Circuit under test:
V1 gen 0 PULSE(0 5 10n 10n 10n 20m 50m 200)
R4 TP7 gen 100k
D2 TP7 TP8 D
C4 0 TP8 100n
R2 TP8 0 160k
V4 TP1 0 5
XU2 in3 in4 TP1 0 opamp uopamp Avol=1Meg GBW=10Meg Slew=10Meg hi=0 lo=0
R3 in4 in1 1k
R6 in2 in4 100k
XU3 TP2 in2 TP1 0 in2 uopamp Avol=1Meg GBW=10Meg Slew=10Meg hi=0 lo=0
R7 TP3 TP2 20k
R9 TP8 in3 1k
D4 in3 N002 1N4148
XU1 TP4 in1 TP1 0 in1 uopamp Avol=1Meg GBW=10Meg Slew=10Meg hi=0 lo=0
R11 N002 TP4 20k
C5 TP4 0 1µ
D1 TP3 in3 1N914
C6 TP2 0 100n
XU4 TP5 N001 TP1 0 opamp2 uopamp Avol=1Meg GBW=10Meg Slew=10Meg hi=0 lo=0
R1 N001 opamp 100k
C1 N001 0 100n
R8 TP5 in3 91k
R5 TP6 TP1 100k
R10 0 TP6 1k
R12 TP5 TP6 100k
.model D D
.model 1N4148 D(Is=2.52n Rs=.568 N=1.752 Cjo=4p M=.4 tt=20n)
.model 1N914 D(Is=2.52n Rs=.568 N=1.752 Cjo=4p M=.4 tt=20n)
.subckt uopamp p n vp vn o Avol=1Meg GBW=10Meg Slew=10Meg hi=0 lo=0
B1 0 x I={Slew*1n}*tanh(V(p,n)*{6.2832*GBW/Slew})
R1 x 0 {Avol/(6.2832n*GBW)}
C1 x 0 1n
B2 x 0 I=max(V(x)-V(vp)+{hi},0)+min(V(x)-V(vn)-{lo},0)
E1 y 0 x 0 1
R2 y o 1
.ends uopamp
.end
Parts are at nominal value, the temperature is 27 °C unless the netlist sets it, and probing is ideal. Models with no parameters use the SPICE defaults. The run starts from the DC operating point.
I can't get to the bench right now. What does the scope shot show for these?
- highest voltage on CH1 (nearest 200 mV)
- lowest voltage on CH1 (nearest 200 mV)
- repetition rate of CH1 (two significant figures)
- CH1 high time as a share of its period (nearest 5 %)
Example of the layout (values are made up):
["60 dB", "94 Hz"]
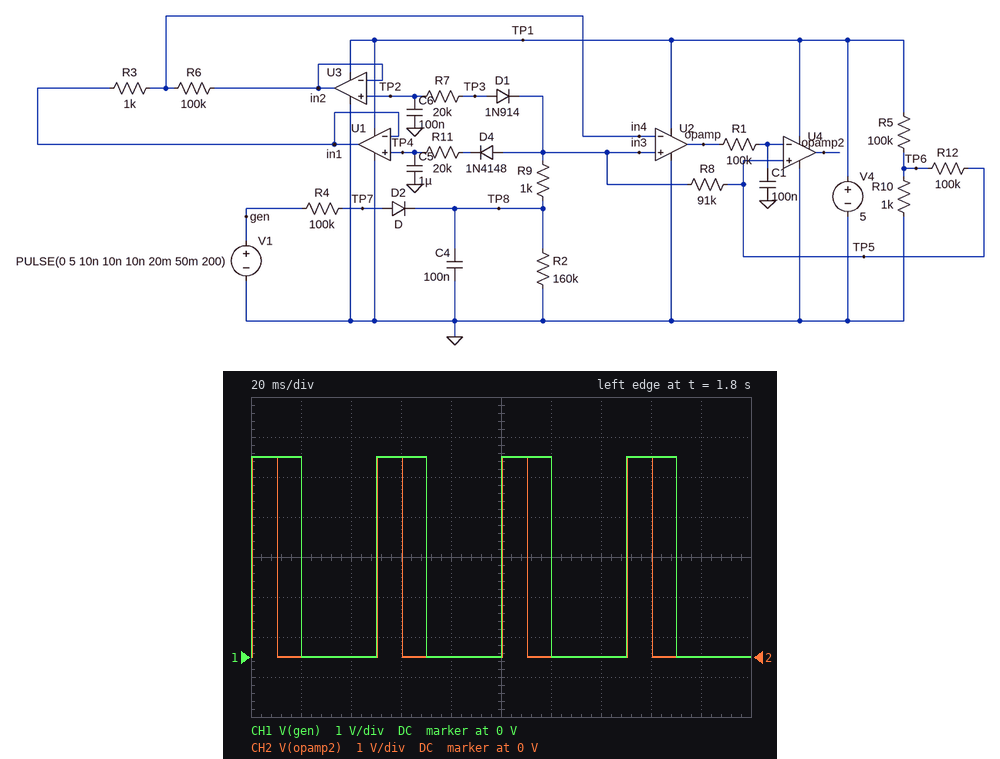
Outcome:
["5.0 V", "0 V", "20 Hz", "40 %"]
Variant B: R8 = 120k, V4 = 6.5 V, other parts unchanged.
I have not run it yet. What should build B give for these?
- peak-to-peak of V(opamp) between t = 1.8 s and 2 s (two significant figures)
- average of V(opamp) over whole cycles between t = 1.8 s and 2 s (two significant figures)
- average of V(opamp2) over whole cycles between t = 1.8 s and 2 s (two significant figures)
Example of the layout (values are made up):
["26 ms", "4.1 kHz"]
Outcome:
["6.5 V", "1.6 V", "1.2 V"]
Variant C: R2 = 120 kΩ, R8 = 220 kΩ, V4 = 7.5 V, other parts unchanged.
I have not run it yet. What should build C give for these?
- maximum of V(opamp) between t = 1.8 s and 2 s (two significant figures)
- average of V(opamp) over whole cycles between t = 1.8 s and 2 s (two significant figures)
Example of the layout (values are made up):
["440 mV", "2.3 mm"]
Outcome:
["7.5 V", "1.9 V"]
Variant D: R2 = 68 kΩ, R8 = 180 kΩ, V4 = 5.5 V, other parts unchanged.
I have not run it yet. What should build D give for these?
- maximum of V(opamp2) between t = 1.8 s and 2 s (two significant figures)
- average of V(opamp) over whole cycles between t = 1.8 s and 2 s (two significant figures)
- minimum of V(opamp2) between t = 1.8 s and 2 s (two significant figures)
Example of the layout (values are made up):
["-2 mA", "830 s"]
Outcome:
["5.5 V", "1.6 V", "-10 mV"]
